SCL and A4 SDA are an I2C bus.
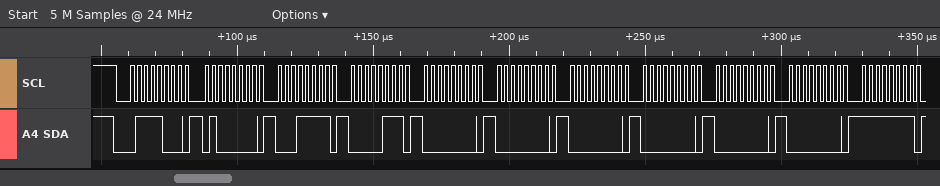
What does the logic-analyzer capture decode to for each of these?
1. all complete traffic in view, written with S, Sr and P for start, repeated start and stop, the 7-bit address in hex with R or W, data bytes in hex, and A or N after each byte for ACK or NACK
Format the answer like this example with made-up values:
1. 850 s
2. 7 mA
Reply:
1. S 3CW A 40 A 1F A 07 A 00 A 00 A 00 A 00 A 00 A 00 A FF A
